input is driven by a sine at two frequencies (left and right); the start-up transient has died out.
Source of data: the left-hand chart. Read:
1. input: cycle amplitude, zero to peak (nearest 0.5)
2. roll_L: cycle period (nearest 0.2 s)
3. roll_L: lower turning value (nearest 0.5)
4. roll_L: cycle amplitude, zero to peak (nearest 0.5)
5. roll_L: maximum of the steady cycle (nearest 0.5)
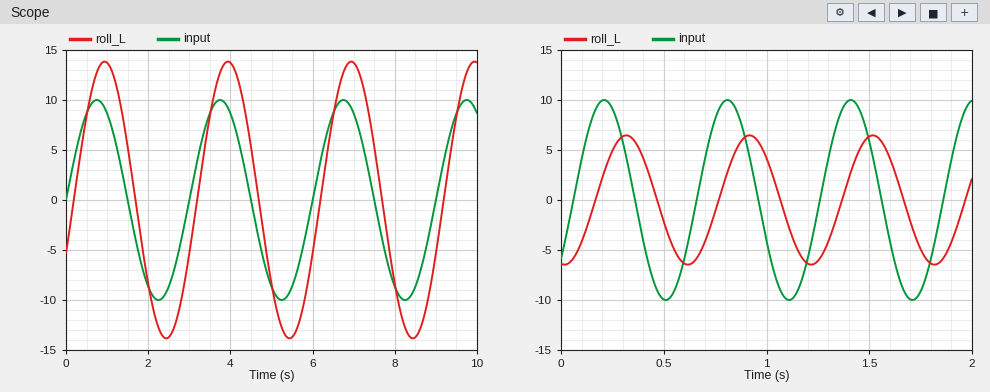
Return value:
10.0
3.0 s
-14.0
14.0
14.0
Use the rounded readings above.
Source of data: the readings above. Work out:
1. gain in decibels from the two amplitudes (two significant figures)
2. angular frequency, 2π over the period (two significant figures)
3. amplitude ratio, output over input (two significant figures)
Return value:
2.9 dB
2.1 rad/s
1.4
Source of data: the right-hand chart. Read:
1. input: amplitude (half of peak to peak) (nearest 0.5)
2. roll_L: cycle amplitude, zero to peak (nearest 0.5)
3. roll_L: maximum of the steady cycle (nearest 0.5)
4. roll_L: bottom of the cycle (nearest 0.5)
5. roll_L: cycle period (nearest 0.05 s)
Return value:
10.0
6.5
6.5
-6.5
0.60 s
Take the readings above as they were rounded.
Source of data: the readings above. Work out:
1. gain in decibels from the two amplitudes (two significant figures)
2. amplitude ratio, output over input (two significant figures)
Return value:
-3.7 dB
0.65
